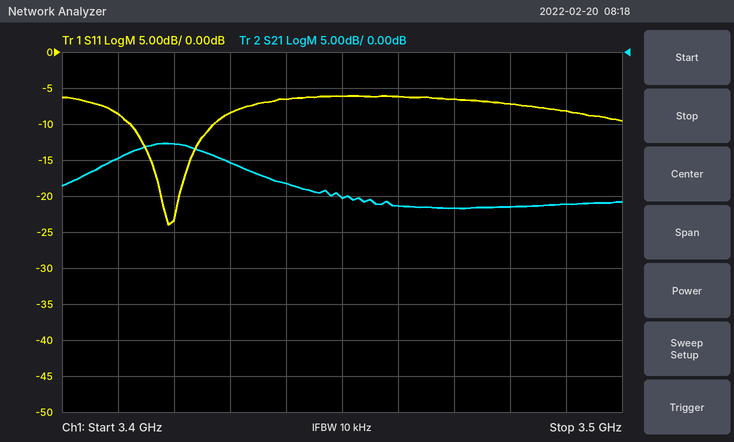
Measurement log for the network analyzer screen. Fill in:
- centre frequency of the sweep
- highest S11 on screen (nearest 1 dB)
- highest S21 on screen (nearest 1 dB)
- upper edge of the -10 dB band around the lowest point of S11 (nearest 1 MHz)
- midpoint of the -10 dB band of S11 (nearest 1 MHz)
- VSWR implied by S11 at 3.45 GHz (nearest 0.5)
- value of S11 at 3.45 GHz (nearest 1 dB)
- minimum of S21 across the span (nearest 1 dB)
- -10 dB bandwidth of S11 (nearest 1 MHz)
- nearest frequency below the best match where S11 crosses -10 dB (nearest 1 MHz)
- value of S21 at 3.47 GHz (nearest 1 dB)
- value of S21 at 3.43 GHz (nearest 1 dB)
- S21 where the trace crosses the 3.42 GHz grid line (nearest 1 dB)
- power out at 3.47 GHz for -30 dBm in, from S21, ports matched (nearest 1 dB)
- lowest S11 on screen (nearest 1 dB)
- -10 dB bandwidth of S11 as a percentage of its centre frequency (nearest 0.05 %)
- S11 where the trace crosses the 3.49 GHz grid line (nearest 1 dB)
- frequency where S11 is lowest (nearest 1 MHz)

3.45 GHz
-6 dB
-13 dB
3.427 GHz
3.420 GHz
3.0
-6 dB
-22 dB
15 MHz
3.412 GHz
-22 dB
-15 dB
-13 dB
-52 dBm
-24 dB
0.45 %
-8 dB
3.419 GHz
